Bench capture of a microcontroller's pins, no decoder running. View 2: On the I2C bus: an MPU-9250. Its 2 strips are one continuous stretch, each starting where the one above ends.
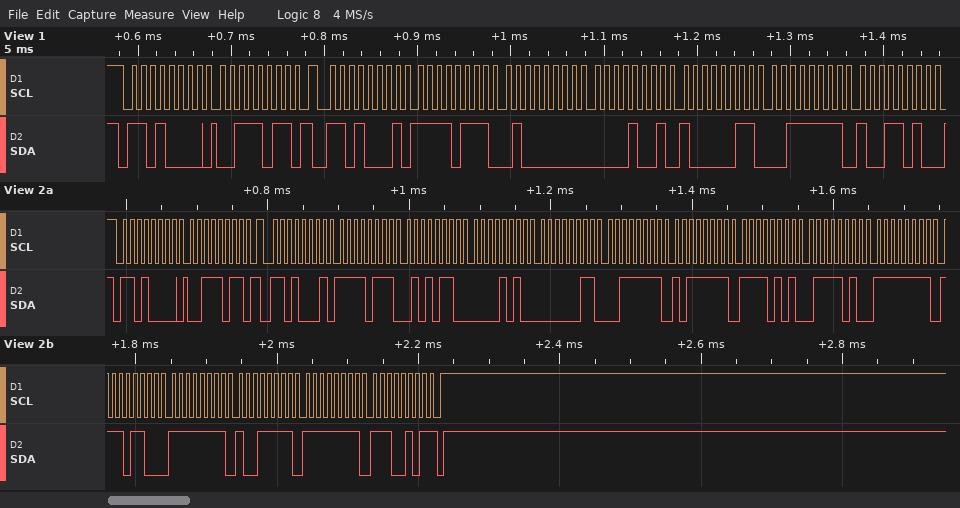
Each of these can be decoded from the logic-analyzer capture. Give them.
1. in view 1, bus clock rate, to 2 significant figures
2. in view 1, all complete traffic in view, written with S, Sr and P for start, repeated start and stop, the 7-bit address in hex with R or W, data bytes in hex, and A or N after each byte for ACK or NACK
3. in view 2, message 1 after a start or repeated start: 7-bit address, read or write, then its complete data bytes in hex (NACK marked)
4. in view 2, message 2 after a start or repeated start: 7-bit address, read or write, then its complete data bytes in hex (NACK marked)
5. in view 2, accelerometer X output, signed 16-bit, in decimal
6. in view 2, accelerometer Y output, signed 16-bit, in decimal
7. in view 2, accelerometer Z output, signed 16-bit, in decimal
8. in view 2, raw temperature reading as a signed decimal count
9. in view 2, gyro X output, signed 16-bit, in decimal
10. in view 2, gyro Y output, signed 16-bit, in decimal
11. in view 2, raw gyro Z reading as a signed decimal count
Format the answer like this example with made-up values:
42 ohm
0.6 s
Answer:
100 kHz
S 68W A 3B A Sr 68R A F7 A 40 A 09 A 83 A 3F A 9A A
0x68 write: 3B
0x68 read: F7 56 0A 03 3F BF F5 7A FF EC FF 9F FF E5 NACK
-2218
2563
16319
-2694
-20
-97
-27
